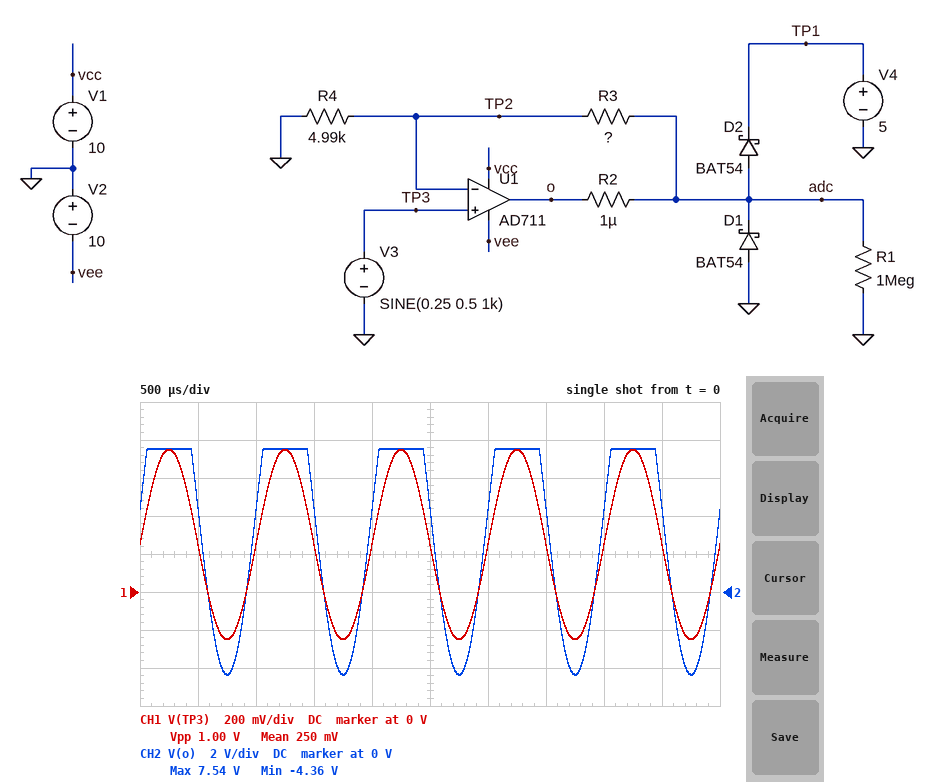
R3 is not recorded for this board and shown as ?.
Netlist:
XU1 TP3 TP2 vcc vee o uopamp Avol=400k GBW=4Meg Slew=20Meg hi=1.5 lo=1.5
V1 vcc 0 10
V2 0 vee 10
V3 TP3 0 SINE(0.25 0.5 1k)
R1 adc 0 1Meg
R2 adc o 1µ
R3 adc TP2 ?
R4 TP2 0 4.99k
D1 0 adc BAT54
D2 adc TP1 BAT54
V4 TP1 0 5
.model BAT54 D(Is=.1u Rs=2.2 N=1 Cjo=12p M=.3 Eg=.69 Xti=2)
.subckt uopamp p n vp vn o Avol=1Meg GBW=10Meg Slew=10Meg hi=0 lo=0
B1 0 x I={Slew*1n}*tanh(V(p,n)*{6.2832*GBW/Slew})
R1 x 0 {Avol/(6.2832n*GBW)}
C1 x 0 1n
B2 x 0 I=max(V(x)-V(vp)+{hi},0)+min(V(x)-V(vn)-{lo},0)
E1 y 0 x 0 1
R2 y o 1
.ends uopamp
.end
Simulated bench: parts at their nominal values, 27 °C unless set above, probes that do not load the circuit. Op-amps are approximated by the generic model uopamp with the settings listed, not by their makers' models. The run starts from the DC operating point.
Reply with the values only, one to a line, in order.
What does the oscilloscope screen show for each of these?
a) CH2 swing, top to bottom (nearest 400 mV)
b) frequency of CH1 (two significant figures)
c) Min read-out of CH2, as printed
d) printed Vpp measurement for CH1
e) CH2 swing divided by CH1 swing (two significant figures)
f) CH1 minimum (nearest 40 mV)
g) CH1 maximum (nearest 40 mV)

12.0 V
1.0 kHz
-4.36 V
1.00 V
12
-240 mV
760 mV
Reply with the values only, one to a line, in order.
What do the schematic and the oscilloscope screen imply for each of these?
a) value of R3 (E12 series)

82 kΩ
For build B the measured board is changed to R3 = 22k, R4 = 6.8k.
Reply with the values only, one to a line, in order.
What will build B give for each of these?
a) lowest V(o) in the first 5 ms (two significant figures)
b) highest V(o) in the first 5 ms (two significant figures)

-1.1 V
3.2 V
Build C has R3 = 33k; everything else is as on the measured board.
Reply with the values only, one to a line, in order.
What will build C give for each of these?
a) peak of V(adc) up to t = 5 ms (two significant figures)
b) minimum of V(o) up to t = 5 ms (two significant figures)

5.7 V
-1.9 V
